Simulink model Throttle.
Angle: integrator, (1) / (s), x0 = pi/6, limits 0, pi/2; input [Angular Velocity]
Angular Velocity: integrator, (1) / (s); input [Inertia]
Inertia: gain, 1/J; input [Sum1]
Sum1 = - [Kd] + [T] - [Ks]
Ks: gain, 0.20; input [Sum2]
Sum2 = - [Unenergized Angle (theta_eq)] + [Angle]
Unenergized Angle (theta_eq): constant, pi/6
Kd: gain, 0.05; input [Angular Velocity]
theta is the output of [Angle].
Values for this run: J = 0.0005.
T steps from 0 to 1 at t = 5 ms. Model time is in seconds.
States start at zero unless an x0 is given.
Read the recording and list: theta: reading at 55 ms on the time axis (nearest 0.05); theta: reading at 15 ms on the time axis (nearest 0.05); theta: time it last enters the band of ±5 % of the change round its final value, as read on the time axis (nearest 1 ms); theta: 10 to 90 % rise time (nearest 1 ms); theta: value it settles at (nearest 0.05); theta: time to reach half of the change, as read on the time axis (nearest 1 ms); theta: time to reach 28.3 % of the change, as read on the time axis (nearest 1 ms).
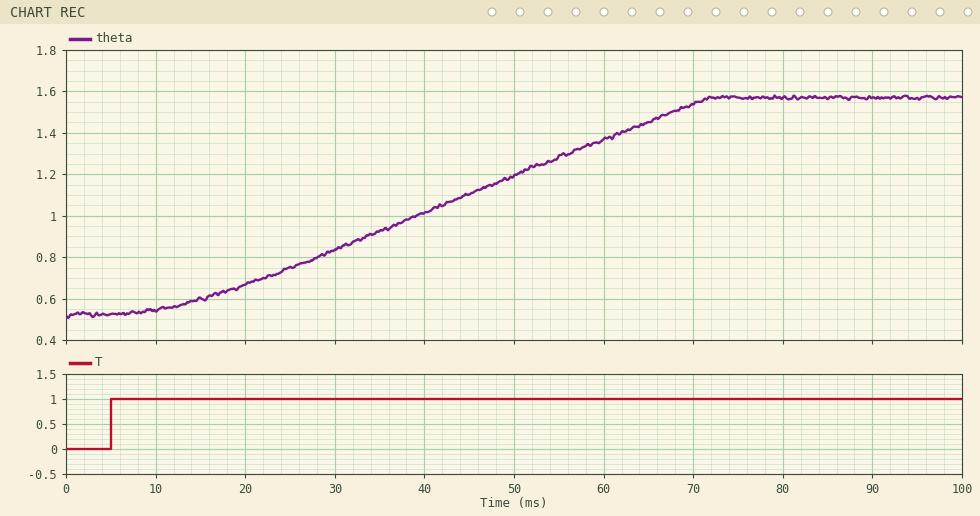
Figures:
1.30
0.60
69 ms
48 ms
1.55
42 ms
29 ms
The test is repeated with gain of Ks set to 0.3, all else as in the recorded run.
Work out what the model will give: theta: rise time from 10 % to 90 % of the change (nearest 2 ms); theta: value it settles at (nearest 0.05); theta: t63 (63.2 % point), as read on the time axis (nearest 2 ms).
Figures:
50 ms
1.55
50 ms
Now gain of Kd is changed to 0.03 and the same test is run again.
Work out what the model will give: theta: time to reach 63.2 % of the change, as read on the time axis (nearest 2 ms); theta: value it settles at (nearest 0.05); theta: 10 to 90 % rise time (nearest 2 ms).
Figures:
40 ms
1.55
34 ms
